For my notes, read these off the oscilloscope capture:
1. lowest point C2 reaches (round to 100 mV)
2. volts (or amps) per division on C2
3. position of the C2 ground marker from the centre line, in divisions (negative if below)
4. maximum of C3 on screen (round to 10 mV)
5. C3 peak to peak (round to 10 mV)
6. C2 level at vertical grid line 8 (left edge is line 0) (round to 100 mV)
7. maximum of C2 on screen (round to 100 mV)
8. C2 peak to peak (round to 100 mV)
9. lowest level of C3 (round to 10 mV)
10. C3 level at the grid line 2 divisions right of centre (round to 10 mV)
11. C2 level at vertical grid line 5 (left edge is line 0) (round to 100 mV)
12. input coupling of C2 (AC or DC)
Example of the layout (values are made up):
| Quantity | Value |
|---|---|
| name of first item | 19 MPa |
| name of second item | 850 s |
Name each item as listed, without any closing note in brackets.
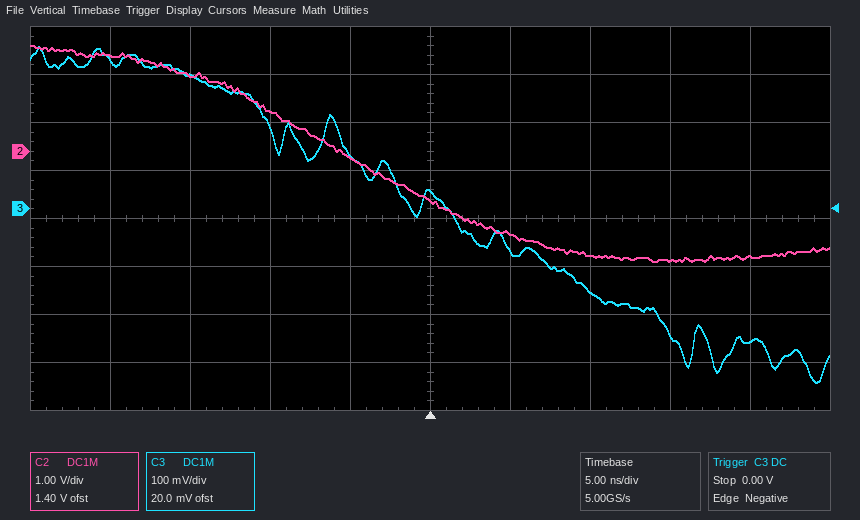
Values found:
| Quantity | Value |
|---|---|
| lowest point C2 reaches | -2.3 V |
| volts (or amps) per division on C2 | 1 V |
| position of the C2 ground marker from the centre line, in divisions | +1.4 div |
| maximum of C3 on screen | 340 mV |
| C3 peak to peak | 700 mV |
| C2 level at vertical grid line 8 (left edge is line 0) | -2.3 V |
| maximum of C2 on screen | 2.2 V |
| C2 peak to peak | 4.5 V |
| lowest level of C3 | -360 mV |
| C3 level at the grid line 2 divisions right of centre | -170 mV |
| C2 level at vertical grid line 5 (left edge is line 0) | -1.0 V |
| input coupling of C2 | DC |
